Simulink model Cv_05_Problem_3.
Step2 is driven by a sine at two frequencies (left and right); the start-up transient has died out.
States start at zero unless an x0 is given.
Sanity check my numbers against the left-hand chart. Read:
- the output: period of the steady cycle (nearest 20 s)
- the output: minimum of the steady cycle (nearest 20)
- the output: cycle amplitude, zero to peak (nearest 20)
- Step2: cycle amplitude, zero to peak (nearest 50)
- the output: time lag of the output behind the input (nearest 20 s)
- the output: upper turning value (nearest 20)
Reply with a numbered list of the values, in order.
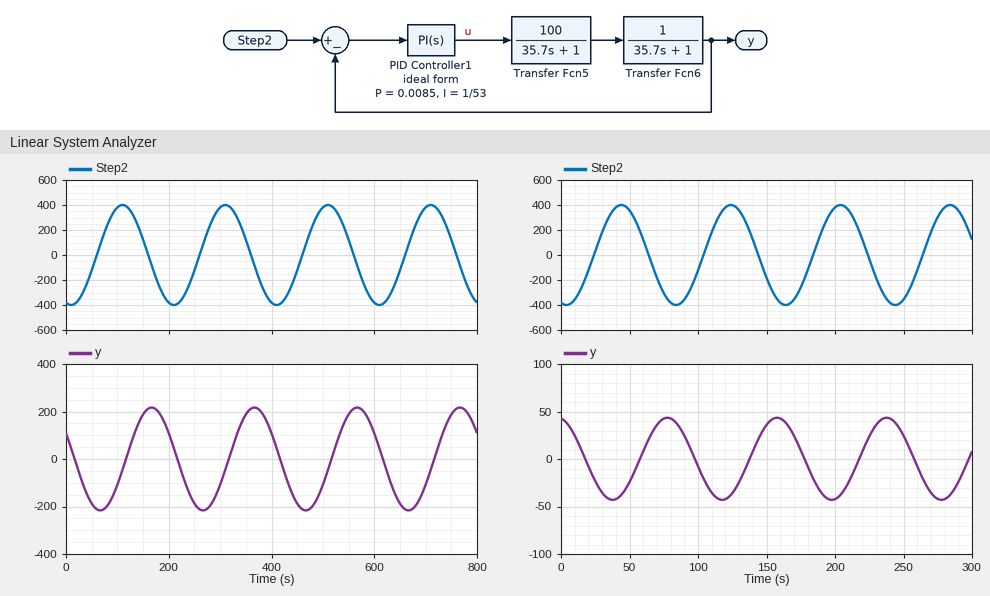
1. 200 s
2. -220
3. 220
4. 400
5. 60 s
6. 220
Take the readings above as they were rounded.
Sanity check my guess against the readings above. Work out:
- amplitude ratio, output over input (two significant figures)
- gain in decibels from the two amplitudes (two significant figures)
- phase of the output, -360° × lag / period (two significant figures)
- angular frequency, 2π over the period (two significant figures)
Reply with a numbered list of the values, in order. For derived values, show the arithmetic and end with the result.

1. 220 / 400 = 0.55
2. 20 log10(220 / 400) = -5.2 dB
3. -360 × 60 / 200 = -110°
4. 2π / 200 = 0.031 rad/s
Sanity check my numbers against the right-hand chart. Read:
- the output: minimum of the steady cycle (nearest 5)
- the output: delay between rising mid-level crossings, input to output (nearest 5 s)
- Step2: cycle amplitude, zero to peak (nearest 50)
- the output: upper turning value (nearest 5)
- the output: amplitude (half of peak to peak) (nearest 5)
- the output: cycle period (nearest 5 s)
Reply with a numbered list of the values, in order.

1. -45
2. 35 s
3. 400
4. 45
5. 45
6. 80 s
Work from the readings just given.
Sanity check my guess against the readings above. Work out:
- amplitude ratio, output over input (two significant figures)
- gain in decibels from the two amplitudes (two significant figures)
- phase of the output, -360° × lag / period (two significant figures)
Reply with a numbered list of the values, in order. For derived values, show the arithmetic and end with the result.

1. 45 / 400 = 0.11
2. 20 log10(45 / 400) = -19 dB
3. -360 × 35 / 80 = -160°
